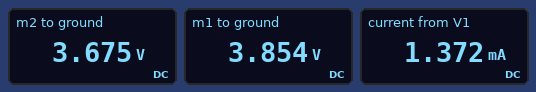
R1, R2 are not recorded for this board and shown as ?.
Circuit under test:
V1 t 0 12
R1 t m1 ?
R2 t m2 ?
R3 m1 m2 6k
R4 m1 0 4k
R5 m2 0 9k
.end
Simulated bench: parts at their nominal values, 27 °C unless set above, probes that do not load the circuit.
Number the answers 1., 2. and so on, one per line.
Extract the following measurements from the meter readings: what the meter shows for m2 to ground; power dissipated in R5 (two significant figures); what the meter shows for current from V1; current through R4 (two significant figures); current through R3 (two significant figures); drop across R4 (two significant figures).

1. 3.675 V
2. 1.5 mW
3. 1.372 mA
4. 960 µA
5. 30 µA
6. 3.9 V
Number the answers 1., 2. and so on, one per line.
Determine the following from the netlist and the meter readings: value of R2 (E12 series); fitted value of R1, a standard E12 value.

1. 22 kΩ
2. 8.2 kΩ
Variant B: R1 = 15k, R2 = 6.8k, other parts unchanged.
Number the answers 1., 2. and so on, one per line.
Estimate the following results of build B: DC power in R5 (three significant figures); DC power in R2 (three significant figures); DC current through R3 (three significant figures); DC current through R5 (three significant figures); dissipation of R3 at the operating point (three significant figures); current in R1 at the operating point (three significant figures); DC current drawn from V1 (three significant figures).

1. 3.43 mW
2. 6.11 mW
3. 331 µA
4. 617 µA
5. 656 µW
6. 562 µA
7. 1.51 mA
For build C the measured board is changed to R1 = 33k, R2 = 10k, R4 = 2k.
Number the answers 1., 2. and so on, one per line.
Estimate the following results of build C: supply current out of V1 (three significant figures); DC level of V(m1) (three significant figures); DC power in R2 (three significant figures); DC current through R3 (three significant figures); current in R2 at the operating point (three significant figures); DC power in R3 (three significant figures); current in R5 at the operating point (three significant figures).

1. 1.14 mA
2. 1.43 V
3. 6.71 mW
4. 396 µA
5. 819 µA
6. 941 µW
7. 423 µA
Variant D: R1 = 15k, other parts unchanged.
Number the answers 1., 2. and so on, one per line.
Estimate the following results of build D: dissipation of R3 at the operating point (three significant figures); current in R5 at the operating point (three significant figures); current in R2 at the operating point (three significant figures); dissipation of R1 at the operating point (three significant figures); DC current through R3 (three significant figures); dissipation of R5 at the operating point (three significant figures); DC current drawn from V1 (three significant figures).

1. 22.8 µW
2. 343 µA
3. 405 µA
4. 5.74 mW
5. 61.6 µA
6. 1.06 mW
7. 1.02 mA
